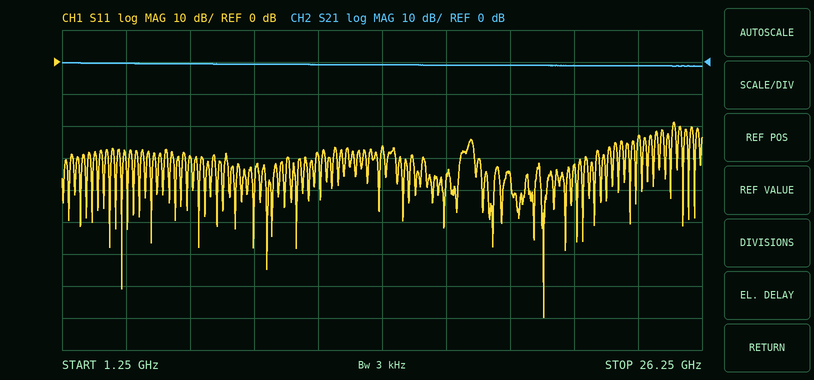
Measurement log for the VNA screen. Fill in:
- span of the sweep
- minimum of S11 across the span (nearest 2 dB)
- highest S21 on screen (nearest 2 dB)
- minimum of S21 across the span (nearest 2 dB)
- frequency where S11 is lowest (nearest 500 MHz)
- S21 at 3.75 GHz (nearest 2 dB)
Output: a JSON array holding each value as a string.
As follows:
["25 GHz", "-80 dB", "0 dB", "-2 dB", "20.0 GHz", "0 dB"]
